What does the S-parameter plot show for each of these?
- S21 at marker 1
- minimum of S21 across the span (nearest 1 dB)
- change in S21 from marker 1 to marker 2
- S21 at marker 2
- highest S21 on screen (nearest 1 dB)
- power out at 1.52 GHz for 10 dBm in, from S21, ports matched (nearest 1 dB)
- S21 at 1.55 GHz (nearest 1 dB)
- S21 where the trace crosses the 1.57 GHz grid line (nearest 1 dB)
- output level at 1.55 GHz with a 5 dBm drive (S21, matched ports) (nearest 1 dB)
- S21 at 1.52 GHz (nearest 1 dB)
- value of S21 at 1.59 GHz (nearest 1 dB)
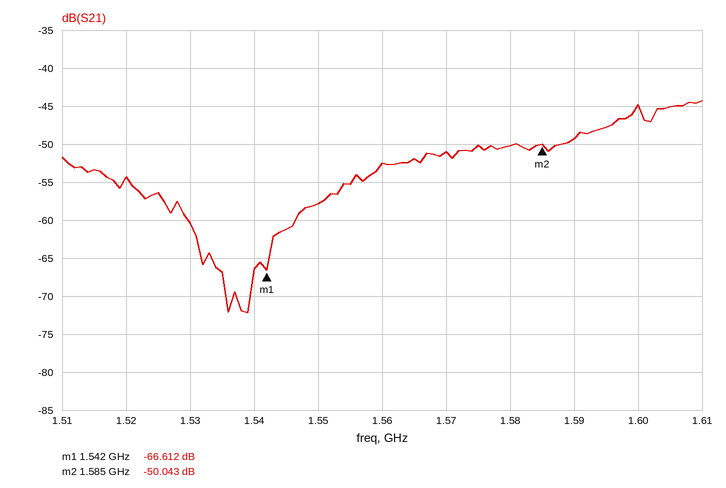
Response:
-66.612 dB
-72 dB
16.569 dB
-50.043 dB
-44 dB
-44 dBm
-58 dB
-51 dB
-53 dBm
-54 dB
-49 dB
